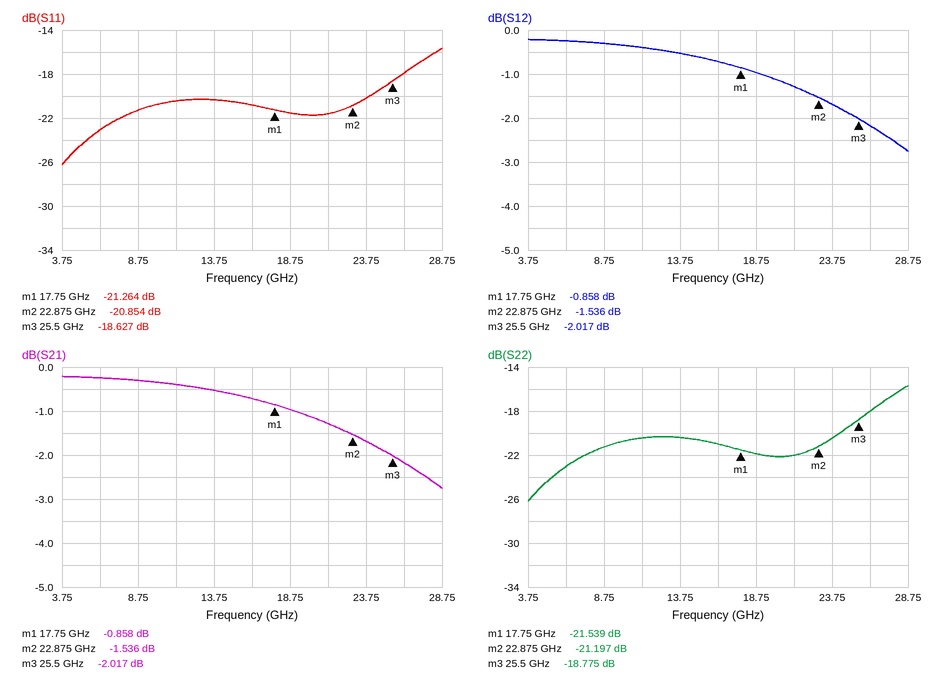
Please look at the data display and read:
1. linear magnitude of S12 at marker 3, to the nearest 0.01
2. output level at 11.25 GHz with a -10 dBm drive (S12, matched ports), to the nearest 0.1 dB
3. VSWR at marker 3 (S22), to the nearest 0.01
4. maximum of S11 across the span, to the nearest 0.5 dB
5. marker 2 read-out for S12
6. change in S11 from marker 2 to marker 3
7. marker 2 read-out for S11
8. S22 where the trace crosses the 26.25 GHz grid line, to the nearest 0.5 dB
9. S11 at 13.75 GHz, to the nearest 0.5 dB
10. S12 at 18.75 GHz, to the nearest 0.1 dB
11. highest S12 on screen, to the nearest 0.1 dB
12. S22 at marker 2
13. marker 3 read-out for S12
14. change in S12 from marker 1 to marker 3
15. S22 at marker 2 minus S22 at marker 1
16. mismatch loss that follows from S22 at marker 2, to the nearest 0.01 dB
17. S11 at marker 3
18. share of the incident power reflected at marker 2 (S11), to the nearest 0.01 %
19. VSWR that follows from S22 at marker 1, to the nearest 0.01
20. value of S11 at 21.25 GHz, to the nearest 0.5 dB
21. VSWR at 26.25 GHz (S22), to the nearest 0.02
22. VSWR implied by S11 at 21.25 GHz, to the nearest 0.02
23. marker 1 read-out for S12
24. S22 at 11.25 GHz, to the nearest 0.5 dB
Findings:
0.79
-10.4 dBm
1.26
-15.5 dB
-1.536 dB
2.227 dB
-20.854 dB
-18.0 dB
-20.5 dB
-1.0 dB
-0.2 dB
-21.197 dB
-2.017 dB
-1.159 dB
0.342 dB
0.03 dB
-18.627 dB
0.82 %
1.18
-21.5 dB
1.28
1.18
-0.858 dB
-20.5 dB
